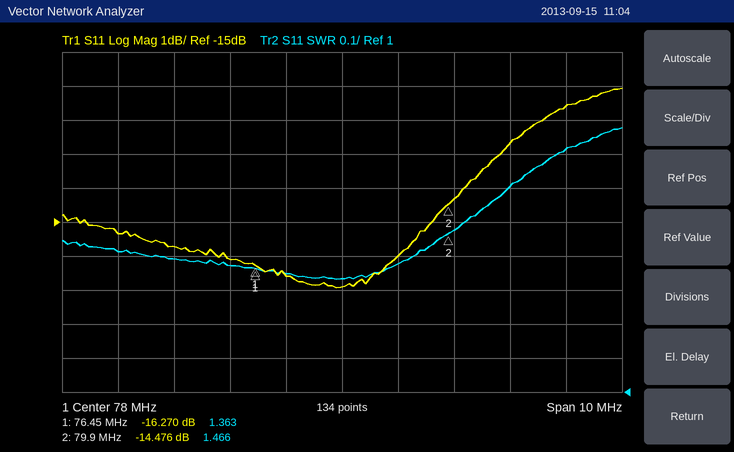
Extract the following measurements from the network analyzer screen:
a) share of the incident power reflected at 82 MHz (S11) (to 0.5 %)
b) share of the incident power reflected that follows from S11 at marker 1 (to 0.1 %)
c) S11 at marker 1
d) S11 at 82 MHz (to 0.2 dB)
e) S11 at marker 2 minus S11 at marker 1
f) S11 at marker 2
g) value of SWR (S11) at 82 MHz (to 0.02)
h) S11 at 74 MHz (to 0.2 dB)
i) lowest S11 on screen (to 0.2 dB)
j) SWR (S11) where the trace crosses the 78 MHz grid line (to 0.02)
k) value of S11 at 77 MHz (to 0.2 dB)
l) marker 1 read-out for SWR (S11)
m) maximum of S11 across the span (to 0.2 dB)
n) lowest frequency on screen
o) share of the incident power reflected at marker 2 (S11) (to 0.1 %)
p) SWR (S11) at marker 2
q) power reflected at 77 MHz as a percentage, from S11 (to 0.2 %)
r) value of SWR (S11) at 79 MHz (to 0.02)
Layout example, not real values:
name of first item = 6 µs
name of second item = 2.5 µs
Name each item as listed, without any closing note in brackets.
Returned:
share of the incident power reflected at 82 MHz (S11) = 7.0 %
share of the incident power reflected that follows from S11 at marker 1 = 2.4 %
S11 at marker 1 = -16.270 dB
S11 at 82 MHz = -11.6 dB
S11 at marker 2 minus S11 at marker 1 = 1.794 dB
S11 at marker 2 = -14.476 dB
value of SWR (S11) at 82 MHz = 1.72
S11 at 74 MHz = -15.4 dB
lowest S11 on screen = -17.0 dB
SWR (S11) where the trace crosses the 78 MHz grid line = 1.34
value of S11 at 77 MHz = -16.6 dB
marker 1 read-out for SWR = 1.363
maximum of S11 across the span = -11.0 dB
lowest frequency on screen = 73 MHz
share of the incident power reflected at marker 2 (S11) = 3.6 %
SWR (S11) at marker 2 = 1.466
power reflected at 77 MHz as a percentage, from S11 = 2.2 %
value of SWR (S11) at 79 MHz = 1.38
